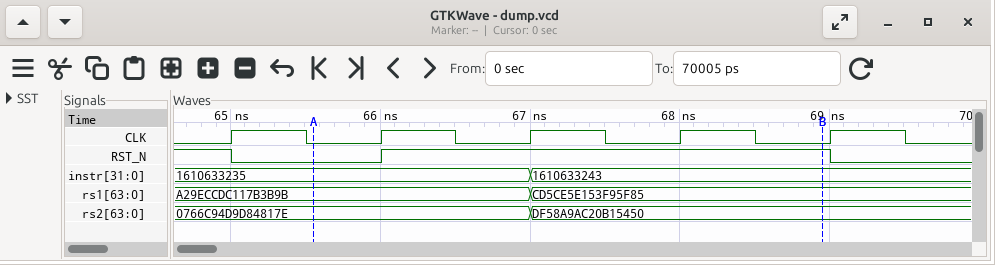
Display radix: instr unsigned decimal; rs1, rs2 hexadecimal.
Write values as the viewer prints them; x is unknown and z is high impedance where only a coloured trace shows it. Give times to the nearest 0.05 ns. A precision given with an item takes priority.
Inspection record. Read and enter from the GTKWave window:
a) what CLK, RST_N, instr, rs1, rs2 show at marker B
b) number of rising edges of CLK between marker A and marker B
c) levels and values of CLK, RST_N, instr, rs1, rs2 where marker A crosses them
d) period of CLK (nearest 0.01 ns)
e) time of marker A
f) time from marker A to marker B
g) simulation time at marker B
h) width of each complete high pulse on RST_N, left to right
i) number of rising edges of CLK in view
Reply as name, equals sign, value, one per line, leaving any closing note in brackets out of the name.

what CLK, RST_N, instr, rs1, rs2 show at marker B = CLK=0, RST_N=1, instr=1610633243, rs1=CD5CE5E153F95F85, rs2=DF58A9AC20B15450
number of rising edges of CLK between marker A and marker B = 3
levels and values of CLK, RST_N, instr, rs1, rs2 where marker A crosses them = CLK=0, RST_N=0, instr=1610633235, rs1=A29ECCDC117B3B9B, rs2=0766C94D9D84817E
period of CLK = 1 ns
time of marker A = 65.55 ns
time from marker A to marker B = 3.4 ns
simulation time at marker B = 68.95 ns
width of each complete high pulse on RST_N, left to right = 3 ns
number of rising edges of CLK in view = 5
